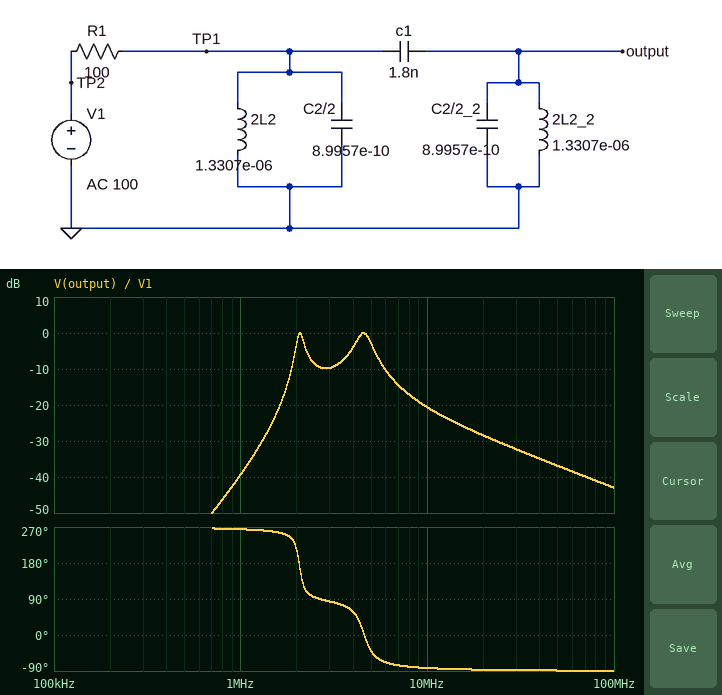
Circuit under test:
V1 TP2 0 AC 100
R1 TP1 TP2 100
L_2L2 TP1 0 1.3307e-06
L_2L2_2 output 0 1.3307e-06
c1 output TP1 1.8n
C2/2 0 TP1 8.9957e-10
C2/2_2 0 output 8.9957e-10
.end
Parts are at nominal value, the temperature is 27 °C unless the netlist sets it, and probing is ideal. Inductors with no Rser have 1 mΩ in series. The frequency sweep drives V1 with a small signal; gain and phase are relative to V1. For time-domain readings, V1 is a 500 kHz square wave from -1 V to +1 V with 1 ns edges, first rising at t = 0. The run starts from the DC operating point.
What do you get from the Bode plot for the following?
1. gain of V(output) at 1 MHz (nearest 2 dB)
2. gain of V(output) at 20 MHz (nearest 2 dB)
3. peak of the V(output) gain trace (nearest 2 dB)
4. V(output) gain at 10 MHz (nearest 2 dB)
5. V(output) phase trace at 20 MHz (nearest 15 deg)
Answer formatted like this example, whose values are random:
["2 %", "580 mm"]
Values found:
["-40 dB", "-28 dB", "0 dB", "-20 dB", "-90 deg"]
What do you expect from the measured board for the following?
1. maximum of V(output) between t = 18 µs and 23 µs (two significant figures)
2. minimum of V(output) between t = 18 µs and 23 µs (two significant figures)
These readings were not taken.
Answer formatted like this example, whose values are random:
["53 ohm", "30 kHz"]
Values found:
["360 mV", "-360 mV"]
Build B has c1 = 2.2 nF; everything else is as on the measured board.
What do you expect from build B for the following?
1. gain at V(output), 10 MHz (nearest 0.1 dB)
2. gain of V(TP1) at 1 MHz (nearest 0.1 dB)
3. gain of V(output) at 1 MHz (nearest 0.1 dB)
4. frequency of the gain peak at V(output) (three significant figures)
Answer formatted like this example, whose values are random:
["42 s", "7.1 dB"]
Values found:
["-20.4 dB", "-19.9 dB", "-37.1 dB", "1.91 MHz"]
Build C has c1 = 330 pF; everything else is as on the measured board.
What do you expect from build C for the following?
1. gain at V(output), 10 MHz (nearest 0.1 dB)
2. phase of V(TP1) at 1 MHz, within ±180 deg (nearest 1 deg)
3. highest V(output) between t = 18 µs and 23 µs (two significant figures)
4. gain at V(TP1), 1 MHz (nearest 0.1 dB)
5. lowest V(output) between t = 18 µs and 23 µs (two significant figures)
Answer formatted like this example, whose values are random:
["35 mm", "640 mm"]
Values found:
["-25.5 dB", "85 deg", "350 mV", "-21.0 dB", "-350 mV"]
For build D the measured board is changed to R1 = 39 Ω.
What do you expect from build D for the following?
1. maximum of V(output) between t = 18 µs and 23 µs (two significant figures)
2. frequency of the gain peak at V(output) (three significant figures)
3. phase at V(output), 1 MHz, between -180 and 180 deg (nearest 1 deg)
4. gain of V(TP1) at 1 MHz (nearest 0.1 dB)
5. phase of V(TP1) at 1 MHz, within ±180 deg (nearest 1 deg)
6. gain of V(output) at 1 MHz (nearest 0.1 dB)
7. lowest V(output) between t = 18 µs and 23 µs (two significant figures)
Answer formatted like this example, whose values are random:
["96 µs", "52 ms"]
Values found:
["630 mV", "2.19 MHz", "-104 deg", "-12.2 dB", "76 deg", "-31.4 dB", "-630 mV"]
